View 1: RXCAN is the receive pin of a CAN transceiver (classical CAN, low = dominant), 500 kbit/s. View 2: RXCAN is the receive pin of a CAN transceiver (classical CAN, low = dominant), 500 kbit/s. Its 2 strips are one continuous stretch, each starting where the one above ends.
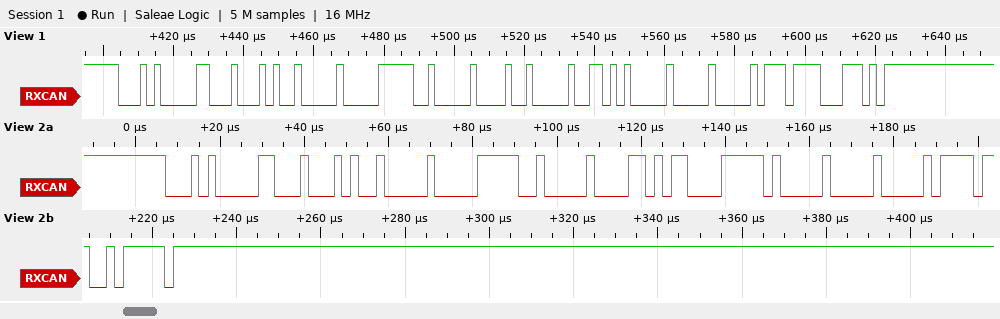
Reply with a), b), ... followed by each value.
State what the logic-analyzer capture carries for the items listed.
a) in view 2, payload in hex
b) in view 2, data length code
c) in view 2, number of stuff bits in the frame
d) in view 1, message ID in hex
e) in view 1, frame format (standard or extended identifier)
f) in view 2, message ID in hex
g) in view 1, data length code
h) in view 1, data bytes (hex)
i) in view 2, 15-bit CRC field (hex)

a) A4 00 F4 01 AC 3F 00 00
b) 8
c) 9
d) 0x141
e) standard
f) 0x141
g) 8
h) A4 00 F4 01 20 35 00 00
i) 0x7B2F
